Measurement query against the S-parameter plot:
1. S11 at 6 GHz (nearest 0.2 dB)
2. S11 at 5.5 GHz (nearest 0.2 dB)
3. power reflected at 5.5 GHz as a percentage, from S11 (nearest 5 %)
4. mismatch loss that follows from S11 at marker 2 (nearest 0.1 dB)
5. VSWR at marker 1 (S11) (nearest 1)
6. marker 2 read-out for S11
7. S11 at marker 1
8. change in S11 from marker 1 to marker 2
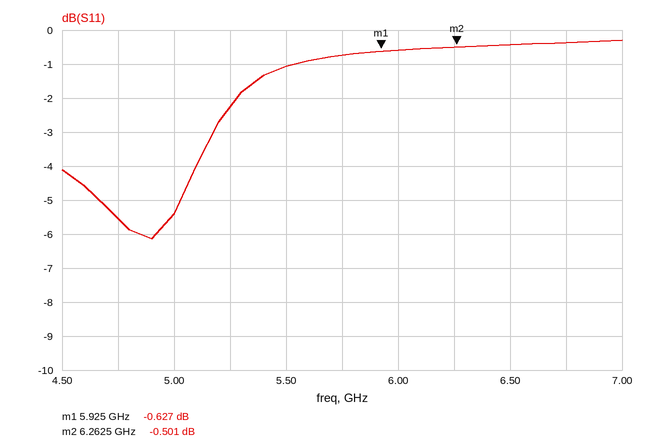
-0.6 dB
-1.0 dB
80 %
9.6 dB
28
-0.501 dB
-0.627 dB
0.126 dB
